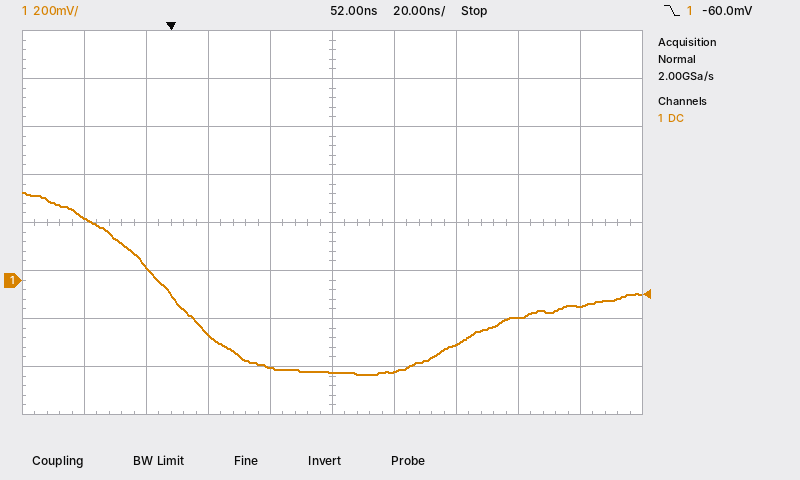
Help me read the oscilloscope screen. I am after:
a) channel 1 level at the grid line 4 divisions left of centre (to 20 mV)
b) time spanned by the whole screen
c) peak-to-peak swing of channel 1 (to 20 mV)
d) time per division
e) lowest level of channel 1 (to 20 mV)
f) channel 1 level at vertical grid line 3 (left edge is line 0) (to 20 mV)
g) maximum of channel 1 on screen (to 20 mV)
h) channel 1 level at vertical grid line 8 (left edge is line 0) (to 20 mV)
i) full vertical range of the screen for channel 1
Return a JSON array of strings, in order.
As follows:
["260 mV", "200 ns", "760 mV", "20 ns", "-400 mV", "-220 mV", "360 mV", "-160 mV", "1.6 V"]
